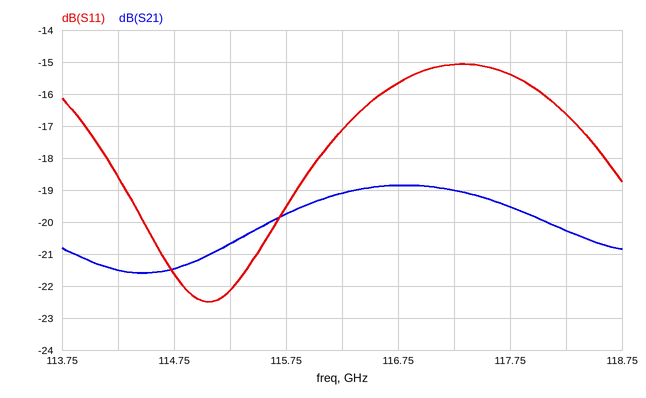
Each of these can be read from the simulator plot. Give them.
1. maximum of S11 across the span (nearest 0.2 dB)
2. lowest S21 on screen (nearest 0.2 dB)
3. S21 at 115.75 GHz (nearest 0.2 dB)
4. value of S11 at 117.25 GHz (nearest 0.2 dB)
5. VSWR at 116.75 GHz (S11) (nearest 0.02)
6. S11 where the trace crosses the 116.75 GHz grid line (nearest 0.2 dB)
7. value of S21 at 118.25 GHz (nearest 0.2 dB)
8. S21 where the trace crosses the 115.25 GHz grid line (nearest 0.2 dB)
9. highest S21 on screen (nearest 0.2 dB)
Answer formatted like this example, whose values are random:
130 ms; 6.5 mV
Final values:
-15.0 dB; -21.6 dB; -19.8 dB; -15.0 dB; 1.40; -15.6 dB; -20.2 dB; -20.6 dB; -18.8 dB
